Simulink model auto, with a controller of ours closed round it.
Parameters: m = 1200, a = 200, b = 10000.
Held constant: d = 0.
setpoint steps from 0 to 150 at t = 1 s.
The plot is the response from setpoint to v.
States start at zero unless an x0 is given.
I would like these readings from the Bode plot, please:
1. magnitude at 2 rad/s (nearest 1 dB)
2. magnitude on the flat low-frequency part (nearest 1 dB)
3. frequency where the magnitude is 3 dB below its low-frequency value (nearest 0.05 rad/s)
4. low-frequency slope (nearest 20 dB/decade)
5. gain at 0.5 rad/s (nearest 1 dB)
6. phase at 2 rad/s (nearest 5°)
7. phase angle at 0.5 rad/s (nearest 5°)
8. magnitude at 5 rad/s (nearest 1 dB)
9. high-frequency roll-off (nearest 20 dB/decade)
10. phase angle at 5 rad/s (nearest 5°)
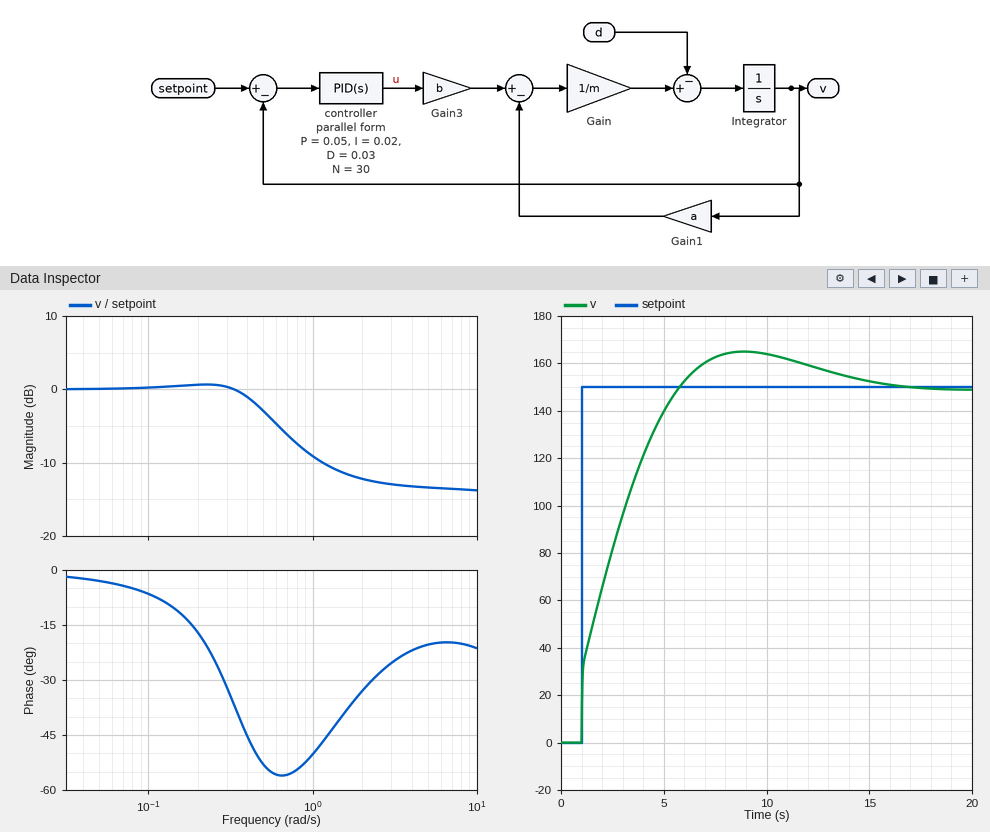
-12 dB
0 dB
0.50 rad/s
0 dB/decade
-3 dB
-35°
-55°
-13 dB
0 dB/decade
-20°
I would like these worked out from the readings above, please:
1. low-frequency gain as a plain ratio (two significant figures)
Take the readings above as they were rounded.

1.0
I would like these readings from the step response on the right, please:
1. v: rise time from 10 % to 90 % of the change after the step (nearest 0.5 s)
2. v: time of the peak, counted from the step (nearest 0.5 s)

3.5 s
8.0 s
